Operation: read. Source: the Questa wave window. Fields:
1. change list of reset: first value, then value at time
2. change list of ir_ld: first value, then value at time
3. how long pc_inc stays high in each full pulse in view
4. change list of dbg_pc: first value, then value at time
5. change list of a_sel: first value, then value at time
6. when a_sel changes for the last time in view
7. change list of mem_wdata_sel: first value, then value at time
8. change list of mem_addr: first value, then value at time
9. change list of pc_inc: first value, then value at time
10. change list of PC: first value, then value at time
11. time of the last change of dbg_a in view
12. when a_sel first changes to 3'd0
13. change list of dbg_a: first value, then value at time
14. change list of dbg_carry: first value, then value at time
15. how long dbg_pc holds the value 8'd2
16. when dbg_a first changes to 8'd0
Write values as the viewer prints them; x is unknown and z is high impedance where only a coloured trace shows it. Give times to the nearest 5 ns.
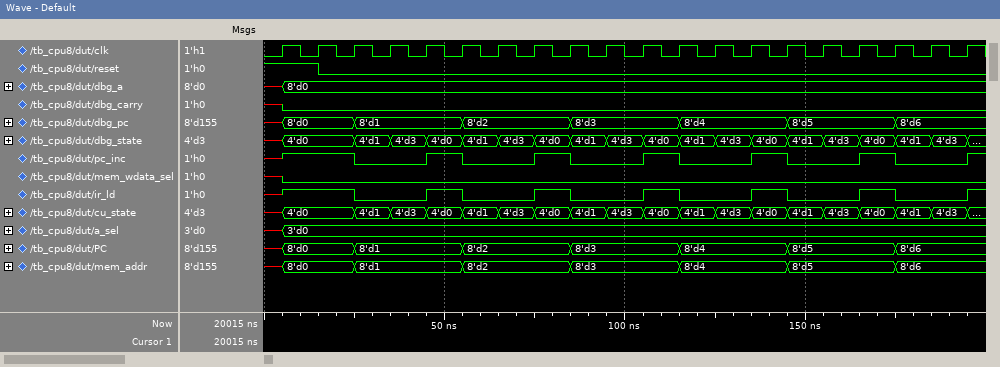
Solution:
1, 0 at 15 ns
x, 1 at 5 ns, 0 at 25 ns, 1 at 45 ns, 0 at 55 ns, 1 at 75 ns, 0 at 85 ns, 1 at 105 ns, 0 at 115 ns, 1 at 135 ns, 0 at 145 ns, 1 at 165 ns, 0 at 175 ns, 1 at 195 ns
10 ns, 10 ns, 10 ns, 10 ns, 10 ns
x, 8'd0 at 5 ns, 8'd1 at 25 ns, 8'd2 at 55 ns, 8'd3 at 85 ns, 8'd4 at 115 ns, 8'd5 at 145 ns, 8'd6 at 175 ns
x, 3'd0 at 5 ns
5 ns
x, 0 at 5 ns
x, 8'd0 at 5 ns, 8'd1 at 25 ns, 8'd2 at 55 ns, 8'd3 at 85 ns, 8'd4 at 115 ns, 8'd5 at 145 ns, 8'd6 at 175 ns
x, 1 at 5 ns, 0 at 25 ns, 1 at 45 ns, 0 at 55 ns, 1 at 75 ns, 0 at 85 ns, 1 at 105 ns, 0 at 115 ns, 1 at 135 ns, 0 at 145 ns, 1 at 165 ns, 0 at 175 ns, 1 at 195 ns
x, 8'd0 at 5 ns, 8'd1 at 25 ns, 8'd2 at 55 ns, 8'd3 at 85 ns, 8'd4 at 115 ns, 8'd5 at 145 ns, 8'd6 at 175 ns
5 ns
5 ns
x, 8'd0 at 5 ns
x, 0 at 5 ns
30 ns
5 ns
